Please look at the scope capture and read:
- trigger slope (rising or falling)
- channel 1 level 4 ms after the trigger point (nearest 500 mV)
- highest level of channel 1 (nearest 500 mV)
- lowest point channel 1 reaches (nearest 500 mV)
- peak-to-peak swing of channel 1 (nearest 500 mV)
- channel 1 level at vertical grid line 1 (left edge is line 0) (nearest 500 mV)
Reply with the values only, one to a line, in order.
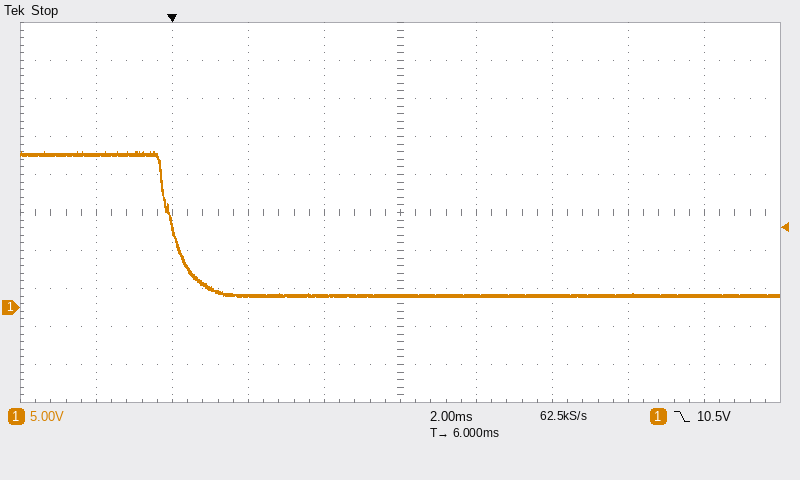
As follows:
falling
1.5 V
20.5 V
1.5 V
19.0 V
20.0 V
